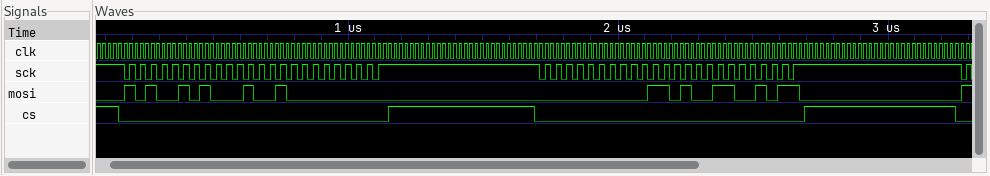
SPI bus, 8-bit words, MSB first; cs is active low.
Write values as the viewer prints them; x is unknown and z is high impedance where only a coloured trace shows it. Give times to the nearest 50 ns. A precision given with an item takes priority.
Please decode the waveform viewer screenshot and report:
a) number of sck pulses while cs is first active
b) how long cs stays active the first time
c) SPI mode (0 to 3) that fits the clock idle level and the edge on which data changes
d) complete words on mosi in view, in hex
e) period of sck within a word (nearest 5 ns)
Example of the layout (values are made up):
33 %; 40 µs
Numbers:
24; 1000 ns; 3; A5, 12, 00, 00, 34, CB; 40 ns
